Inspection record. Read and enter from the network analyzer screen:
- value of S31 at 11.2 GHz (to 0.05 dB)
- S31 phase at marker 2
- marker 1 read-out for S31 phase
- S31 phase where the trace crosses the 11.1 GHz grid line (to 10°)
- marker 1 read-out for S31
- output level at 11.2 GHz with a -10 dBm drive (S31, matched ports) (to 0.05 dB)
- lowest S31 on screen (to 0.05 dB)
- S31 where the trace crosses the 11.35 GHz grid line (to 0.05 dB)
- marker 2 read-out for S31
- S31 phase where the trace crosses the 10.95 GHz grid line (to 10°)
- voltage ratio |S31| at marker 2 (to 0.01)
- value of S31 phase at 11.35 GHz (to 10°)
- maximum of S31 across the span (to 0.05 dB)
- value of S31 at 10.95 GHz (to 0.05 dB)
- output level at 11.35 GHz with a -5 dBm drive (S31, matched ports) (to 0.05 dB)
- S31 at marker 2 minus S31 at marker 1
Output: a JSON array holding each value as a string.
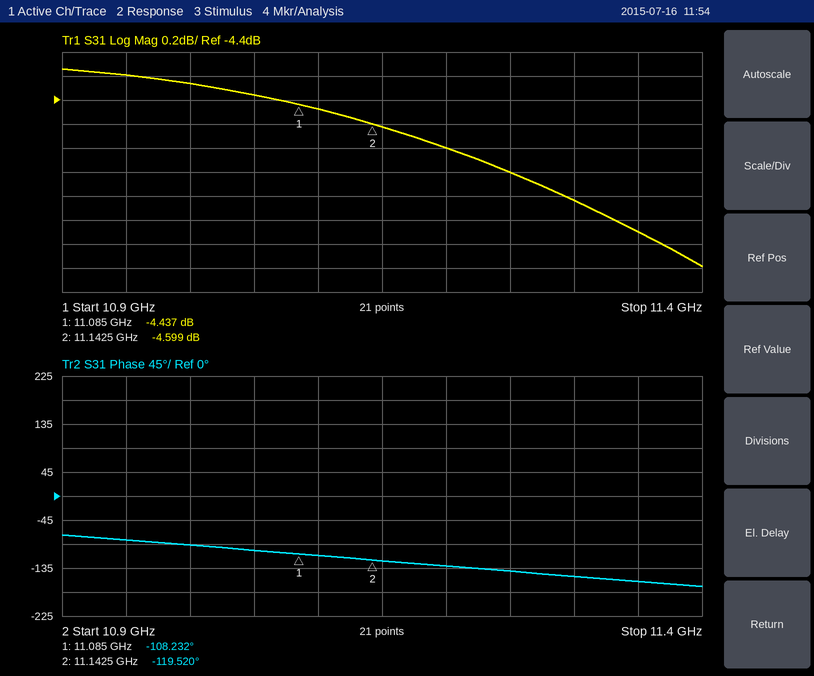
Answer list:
["-4.80 dB", "-119.520°", "-108.232°", "-110°", "-4.437 dB", "-14.80 dBm", "-5.80 dB", "-5.50 dB", "-4.599 dB", "-80°", "0.59", "-160°", "-4.15 dB", "-4.20 dB", "-10.50 dBm", "-0.162 dB"]
